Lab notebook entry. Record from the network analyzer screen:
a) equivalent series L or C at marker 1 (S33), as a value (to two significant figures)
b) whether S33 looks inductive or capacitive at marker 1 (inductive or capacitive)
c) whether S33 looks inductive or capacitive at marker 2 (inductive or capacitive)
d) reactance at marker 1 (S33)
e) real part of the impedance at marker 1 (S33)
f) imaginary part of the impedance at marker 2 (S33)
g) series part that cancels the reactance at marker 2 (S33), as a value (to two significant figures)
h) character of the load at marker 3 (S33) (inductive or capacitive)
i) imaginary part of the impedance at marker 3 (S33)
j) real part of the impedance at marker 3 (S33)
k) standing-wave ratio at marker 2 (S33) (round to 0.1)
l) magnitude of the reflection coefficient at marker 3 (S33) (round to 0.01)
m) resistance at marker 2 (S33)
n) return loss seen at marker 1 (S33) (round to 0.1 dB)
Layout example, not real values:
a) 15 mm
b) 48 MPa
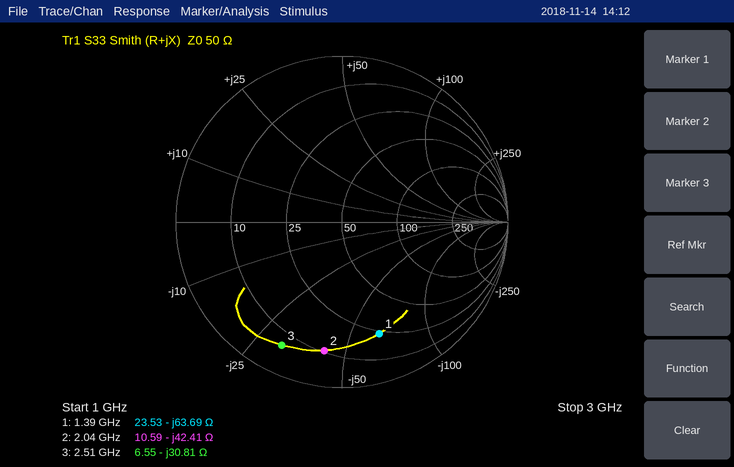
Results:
a) 1.8 pF
b) capacitive
c) capacitive
d) -63.69 Ω
e) 23.53 Ω
f) -42.41 Ω
g) 3.3 nH
h) capacitive
i) -30.81 Ω
j) 6.55 Ω
k) 8.2
l) 0.83
m) 10.59 Ω
n) 3.0 dB
